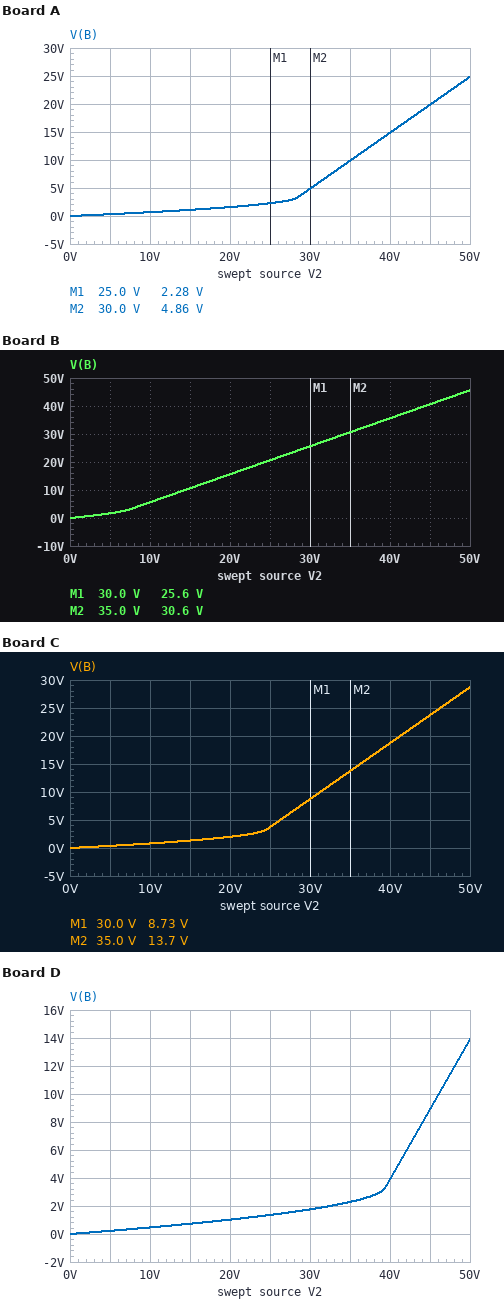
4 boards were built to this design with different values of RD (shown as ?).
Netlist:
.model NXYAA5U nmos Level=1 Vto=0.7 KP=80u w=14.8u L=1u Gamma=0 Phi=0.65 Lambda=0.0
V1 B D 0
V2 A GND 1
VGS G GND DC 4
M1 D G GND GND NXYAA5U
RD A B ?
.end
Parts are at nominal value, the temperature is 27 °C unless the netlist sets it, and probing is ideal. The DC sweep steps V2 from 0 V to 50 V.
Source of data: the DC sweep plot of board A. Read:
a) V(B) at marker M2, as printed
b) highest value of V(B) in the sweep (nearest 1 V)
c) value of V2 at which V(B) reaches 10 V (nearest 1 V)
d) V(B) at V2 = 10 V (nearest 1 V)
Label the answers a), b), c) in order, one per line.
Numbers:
a) 4.86 V
b) 25 V
c) 35 V
d) 1 V
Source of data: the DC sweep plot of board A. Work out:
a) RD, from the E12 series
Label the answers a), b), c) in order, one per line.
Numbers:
a) 3.9 kΩ
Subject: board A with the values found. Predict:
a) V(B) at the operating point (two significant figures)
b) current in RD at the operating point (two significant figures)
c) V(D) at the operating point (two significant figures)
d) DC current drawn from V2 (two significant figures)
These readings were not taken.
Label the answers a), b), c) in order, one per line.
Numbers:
a) 62 mV
b) 240 µA
c) 62 mV
d) 240 µA
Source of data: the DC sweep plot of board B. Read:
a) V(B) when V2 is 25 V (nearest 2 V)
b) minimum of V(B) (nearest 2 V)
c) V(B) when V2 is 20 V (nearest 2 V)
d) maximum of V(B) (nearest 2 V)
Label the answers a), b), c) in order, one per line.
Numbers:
a) 20 V
b) 0 V
c) 16 V
d) 46 V
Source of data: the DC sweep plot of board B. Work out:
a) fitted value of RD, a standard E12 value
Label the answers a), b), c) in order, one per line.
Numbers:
a) 680 Ω
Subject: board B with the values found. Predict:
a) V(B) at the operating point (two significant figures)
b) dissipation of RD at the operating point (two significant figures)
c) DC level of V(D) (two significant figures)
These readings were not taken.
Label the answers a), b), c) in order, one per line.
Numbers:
a) 280 mV
b) 760 µW
c) 280 mV
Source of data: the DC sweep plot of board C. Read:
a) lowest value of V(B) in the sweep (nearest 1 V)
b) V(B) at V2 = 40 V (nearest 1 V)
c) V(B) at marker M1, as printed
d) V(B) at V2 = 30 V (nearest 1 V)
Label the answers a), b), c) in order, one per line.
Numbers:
a) 0 V
b) 19 V
c) 8.73 V
d) 9 V
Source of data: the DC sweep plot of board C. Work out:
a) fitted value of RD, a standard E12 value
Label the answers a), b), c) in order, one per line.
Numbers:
a) 3.3 kΩ
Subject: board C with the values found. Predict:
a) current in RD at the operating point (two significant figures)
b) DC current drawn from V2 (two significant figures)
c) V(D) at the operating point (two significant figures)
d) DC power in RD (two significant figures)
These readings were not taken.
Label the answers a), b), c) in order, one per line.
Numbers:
a) 280 µA
b) 280 µA
c) 73 mV
d) 260 µW
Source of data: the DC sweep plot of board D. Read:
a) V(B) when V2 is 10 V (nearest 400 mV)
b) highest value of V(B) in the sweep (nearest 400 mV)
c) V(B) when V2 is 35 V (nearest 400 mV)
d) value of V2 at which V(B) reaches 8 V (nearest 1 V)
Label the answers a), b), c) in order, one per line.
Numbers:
a) 400 mV
b) 14.0 V
c) 2.4 V
d) 44 V
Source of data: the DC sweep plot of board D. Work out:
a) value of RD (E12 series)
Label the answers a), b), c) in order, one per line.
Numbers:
a) 5.6 kΩ
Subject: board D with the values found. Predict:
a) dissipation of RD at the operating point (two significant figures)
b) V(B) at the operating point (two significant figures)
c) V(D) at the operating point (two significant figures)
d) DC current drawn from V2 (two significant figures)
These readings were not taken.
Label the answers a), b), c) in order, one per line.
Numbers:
a) 160 µW
b) 44 mV
c) 44 mV
d) 170 µA
